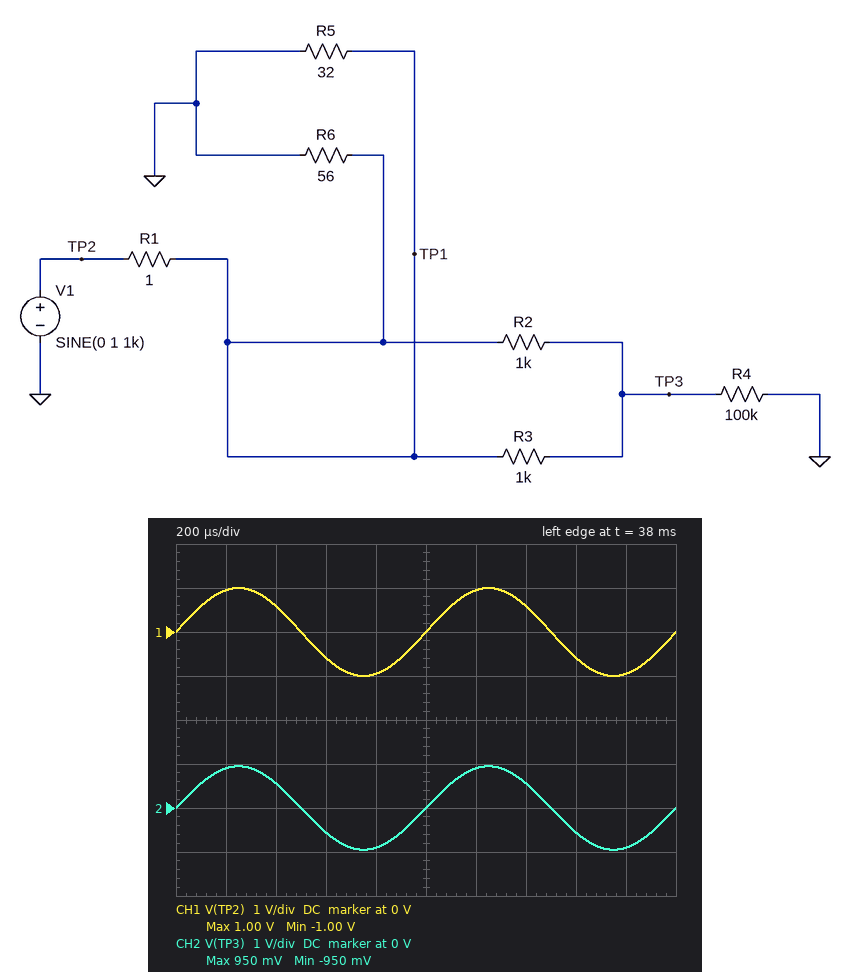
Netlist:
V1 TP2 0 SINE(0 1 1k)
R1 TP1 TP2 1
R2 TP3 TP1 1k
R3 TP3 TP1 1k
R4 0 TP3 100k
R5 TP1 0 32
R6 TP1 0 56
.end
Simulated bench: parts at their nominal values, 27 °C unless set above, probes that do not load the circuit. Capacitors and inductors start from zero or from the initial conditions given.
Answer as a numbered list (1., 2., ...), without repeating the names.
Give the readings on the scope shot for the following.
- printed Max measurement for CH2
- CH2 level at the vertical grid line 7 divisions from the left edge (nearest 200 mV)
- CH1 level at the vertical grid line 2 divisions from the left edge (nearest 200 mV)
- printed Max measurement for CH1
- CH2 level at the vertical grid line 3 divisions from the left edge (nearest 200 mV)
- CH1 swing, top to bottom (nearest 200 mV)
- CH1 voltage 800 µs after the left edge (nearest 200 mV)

1. 950 mV
2. 600 mV
3. 600 mV
4. 1.00 V
5. -600 mV
6. 2.0 V
7. -1.0 V
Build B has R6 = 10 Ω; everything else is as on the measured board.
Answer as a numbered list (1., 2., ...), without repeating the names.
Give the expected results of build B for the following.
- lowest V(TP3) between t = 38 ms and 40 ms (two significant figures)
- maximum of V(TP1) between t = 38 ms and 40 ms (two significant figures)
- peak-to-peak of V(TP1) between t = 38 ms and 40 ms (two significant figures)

1. -880 mV
2. 880 mV
3. 1.8 V
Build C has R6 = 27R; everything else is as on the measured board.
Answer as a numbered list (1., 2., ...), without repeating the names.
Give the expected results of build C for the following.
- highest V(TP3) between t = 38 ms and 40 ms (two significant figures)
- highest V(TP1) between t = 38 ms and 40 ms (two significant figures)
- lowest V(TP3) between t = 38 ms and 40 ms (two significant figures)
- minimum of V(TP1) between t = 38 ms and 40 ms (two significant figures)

1. 930 mV
2. 940 mV
3. -930 mV
4. -940 mV
